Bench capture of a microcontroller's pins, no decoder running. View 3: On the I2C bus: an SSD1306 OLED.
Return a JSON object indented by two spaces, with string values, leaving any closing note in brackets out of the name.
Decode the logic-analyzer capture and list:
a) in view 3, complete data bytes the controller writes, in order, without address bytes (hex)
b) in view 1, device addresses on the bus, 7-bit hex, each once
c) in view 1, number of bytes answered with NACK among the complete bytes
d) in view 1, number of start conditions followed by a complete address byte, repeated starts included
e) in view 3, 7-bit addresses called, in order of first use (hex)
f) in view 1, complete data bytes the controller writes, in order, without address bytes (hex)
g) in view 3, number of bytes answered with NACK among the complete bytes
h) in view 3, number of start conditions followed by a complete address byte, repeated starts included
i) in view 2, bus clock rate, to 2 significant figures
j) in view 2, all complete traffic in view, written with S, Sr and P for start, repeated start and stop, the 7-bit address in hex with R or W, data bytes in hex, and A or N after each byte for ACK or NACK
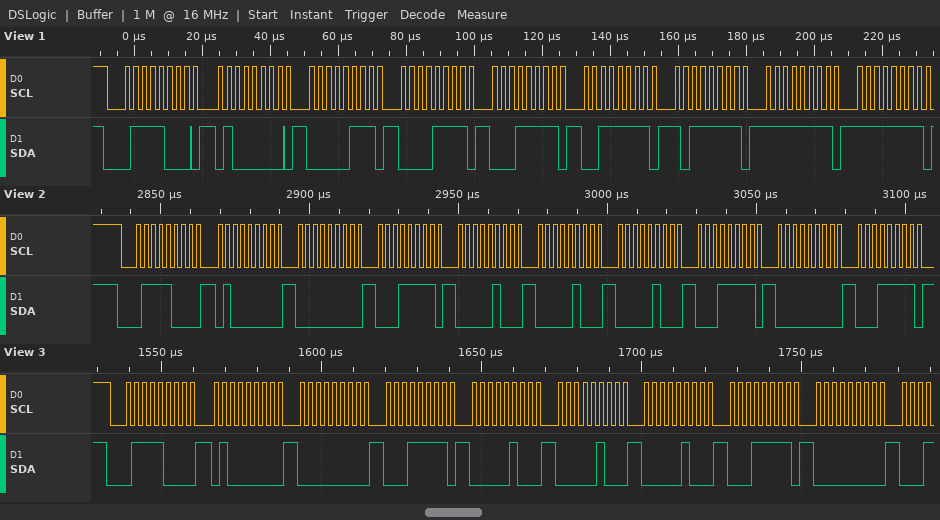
{
  "in view 3, complete data bytes the controller writes, in order, without address bytes": "40 00 1F 04 04 04 1F 00",
  "in view 1, device addresses on the bus, 7-bit hex, each once": "0x3C",
  "in view 1, number of bytes answered with NACK among the complete bytes": "0",
  "in view 1, number of start conditions followed by a complete address byte, repeated starts included": "1",
  "in view 3, 7-bit addresses called, in order of first use": "0x3C",
  "in view 1, complete data bytes the controller writes, in order, without address bytes": "40 07 0F 1F 3F BF FF FF",
  "in view 3, number of bytes answered with NACK among the complete bytes": "0",
  "in view 3, number of start conditions followed by a complete address byte, repeated starts included": "1",
  "in view 2, bus clock rate, to 2 significant figures": "400 kHz",
  "in view 2, all complete traffic in view, written with S, Sr and P for start, repeated start and stop, the 7-bit address in hex with R or W, data bytes in hex, and A or N after each byte for ACK or NACK": "S 3CW A 40 A 00 A 1F A 04 A 04 A 04 A 1F A 00 A 1F A"
}
